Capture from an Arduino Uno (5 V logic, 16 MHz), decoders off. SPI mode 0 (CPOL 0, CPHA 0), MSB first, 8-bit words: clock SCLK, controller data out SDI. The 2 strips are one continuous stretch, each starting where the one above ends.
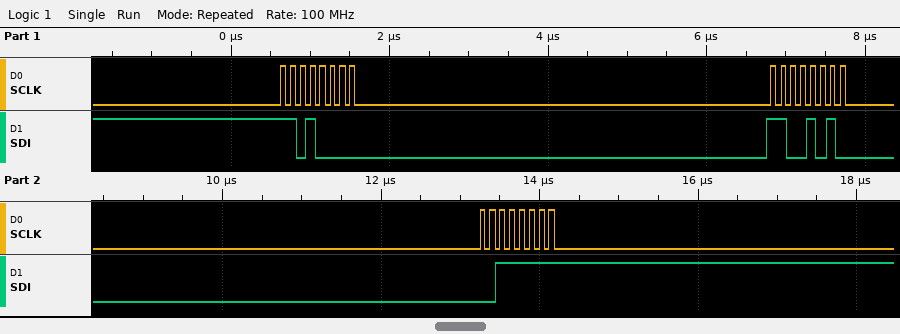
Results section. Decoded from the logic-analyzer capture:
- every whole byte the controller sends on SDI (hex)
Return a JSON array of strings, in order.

["D0 CA 3F"]
